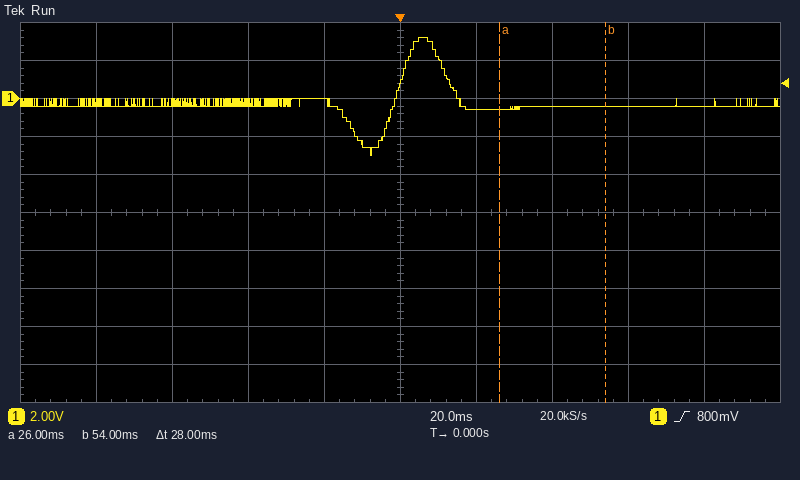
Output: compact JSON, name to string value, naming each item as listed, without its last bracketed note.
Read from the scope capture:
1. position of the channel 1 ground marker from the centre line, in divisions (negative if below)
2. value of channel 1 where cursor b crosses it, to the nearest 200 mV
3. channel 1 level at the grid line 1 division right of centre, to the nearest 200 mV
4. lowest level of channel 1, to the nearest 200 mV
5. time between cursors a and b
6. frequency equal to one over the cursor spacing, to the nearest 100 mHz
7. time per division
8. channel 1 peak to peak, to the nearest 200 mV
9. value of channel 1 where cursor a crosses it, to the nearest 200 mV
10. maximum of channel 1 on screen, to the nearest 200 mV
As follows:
{"position of the channel 1 ground marker from the centre line, in divisions": "+3.0 div", "value of channel 1 where cursor b crosses it, to the nearest 200 mV": "-400 mV", "channel 1 level at the grid line 1 division right of centre, to the nearest 200 mV": "-600 mV", "lowest level of channel 1, to the nearest 200 mV": "-3.0 V", "time between cursors a and b": "28 ms", "frequency equal to one over the cursor spacing, to the nearest 100 mHz": "35.7 Hz", "time per division": "20 ms", "channel 1 peak to peak, to the nearest 200 mV": "6.2 V", "value of channel 1 where cursor a crosses it, to the nearest 200 mV": "-600 mV", "maximum of channel 1 on screen, to the nearest 200 mV": "3.2 V"}
